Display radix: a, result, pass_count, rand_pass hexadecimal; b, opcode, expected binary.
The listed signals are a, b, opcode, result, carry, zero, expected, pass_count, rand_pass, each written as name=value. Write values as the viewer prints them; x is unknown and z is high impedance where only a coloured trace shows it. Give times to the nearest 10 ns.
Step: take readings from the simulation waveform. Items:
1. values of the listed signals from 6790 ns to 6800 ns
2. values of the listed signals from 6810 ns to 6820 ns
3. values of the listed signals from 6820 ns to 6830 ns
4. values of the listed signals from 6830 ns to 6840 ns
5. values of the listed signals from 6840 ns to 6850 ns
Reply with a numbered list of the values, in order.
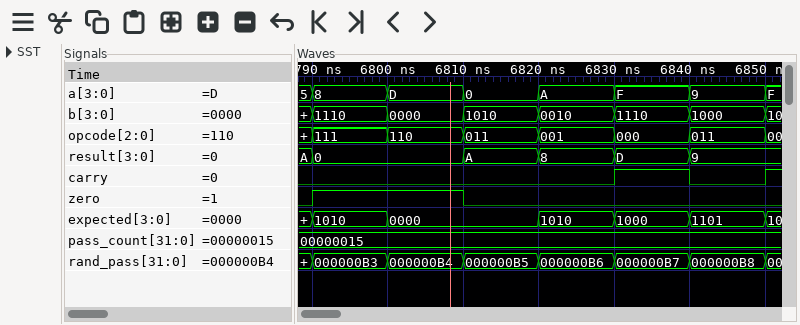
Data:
1. a=8, b=1110, opcode=111, result=0, carry=0, zero=1, expected=1010, pass_count=00000015, rand_pass=000000B3
2. a=0, b=1010, opcode=011, result=A, carry=0, zero=0, expected=0000, pass_count=00000015, rand_pass=000000B5
3. a=A, b=0010, opcode=001, result=8, carry=0, zero=0, expected=1010, pass_count=00000015, rand_pass=000000B6
4. a=F, b=1110, opcode=000, result=D, carry=1, zero=0, expected=1000, pass_count=00000015, rand_pass=000000B7
5. a=9, b=1000, opcode=011, result=9, carry=0, zero=0, expected=1101, pass_count=00000015, rand_pass=000000B8
